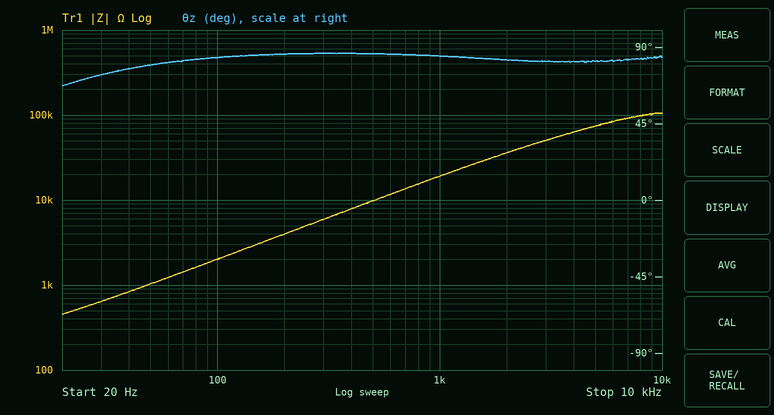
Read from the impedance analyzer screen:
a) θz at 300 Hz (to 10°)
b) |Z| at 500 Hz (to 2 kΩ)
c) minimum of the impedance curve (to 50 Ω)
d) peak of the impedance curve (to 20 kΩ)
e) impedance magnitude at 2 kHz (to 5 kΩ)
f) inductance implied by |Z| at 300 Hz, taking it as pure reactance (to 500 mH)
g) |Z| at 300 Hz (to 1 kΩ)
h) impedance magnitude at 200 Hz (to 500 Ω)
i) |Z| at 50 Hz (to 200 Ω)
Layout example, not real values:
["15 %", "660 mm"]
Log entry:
["90°", "10 kΩ", "450 Ω", "100 kΩ", "35 kΩ", "3.0 H", "6 kΩ", "4.0 kΩ", "1.0 kΩ"]
